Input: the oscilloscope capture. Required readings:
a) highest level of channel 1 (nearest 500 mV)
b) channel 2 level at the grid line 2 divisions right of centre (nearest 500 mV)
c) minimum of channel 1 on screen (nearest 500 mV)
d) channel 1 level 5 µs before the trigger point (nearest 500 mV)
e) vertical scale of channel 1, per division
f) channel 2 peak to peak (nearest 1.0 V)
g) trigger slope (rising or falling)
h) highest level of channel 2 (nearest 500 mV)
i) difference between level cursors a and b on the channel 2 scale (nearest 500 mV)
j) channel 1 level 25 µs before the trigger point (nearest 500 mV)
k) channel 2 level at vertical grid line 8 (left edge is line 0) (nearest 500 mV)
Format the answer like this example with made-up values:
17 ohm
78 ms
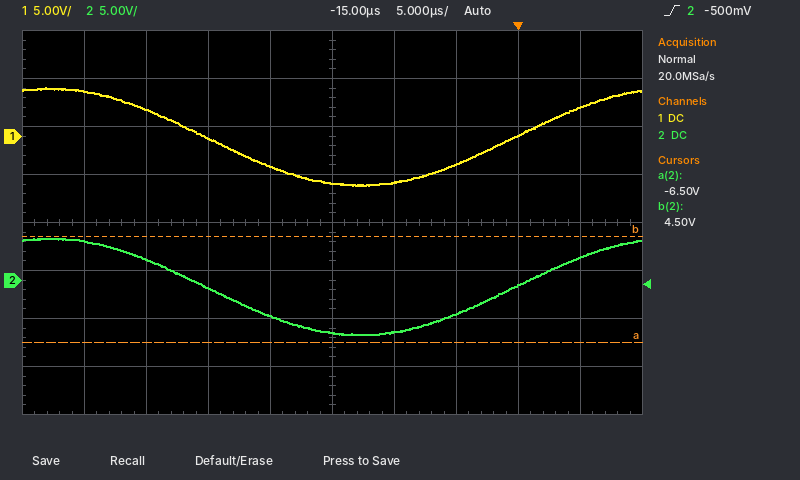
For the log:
5.0 V
-3.5 V
-5.0 V
-3.0 V
5 V
10.0 V
rising
4.5 V
11.0 V
0.0 V
-500 mV
